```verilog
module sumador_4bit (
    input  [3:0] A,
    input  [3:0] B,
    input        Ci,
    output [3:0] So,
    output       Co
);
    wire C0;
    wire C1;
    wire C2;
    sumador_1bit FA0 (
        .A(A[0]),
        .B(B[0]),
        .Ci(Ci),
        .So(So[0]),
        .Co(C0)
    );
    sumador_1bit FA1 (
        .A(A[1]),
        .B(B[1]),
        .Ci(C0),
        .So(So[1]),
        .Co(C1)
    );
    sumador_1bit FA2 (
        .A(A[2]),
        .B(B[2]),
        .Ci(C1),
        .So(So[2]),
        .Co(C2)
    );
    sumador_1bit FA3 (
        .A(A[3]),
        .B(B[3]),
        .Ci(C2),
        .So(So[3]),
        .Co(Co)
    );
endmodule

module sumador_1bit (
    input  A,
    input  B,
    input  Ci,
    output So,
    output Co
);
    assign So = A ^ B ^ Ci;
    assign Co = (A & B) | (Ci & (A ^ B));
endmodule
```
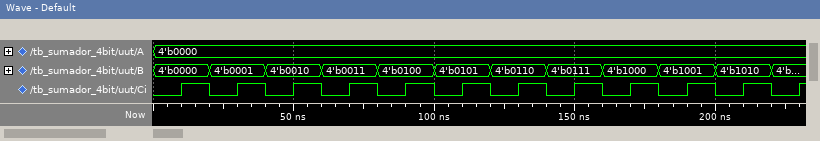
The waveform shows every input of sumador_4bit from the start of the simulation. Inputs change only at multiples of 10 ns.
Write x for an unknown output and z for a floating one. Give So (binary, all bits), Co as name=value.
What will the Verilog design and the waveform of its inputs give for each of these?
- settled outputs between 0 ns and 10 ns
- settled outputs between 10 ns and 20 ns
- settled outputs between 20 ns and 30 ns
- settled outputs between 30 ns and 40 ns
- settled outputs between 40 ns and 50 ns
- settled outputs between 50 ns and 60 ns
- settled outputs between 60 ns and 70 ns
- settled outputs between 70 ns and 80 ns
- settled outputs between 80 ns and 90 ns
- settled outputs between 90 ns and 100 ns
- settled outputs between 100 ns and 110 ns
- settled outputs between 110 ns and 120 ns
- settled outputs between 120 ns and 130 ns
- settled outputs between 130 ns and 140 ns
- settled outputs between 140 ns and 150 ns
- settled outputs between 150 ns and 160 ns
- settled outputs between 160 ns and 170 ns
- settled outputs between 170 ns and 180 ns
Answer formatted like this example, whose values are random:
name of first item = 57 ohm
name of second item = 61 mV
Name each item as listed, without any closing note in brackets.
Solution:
settled outputs between 0 ns and 10 ns = So=0000, Co=0
settled outputs between 10 ns and 20 ns = So=0001, Co=0
settled outputs between 20 ns and 30 ns = So=0001, Co=0
settled outputs between 30 ns and 40 ns = So=0010, Co=0
settled outputs between 40 ns and 50 ns = So=0010, Co=0
settled outputs between 50 ns and 60 ns = So=0011, Co=0
settled outputs between 60 ns and 70 ns = So=0011, Co=0
settled outputs between 70 ns and 80 ns = So=0100, Co=0
settled outputs between 80 ns and 90 ns = So=0100, Co=0
settled outputs between 90 ns and 100 ns = So=0101, Co=0
settled outputs between 100 ns and 110 ns = So=0101, Co=0
settled outputs between 110 ns and 120 ns = So=0110, Co=0
settled outputs between 120 ns and 130 ns = So=0110, Co=0
settled outputs between 130 ns and 140 ns = So=0111, Co=0
settled outputs between 140 ns and 150 ns = So=0111, Co=0
settled outputs between 150 ns and 160 ns = So=1000, Co=0
settled outputs between 160 ns and 170 ns = So=1000, Co=0
settled outputs between 170 ns and 180 ns = So=1001, Co=0
